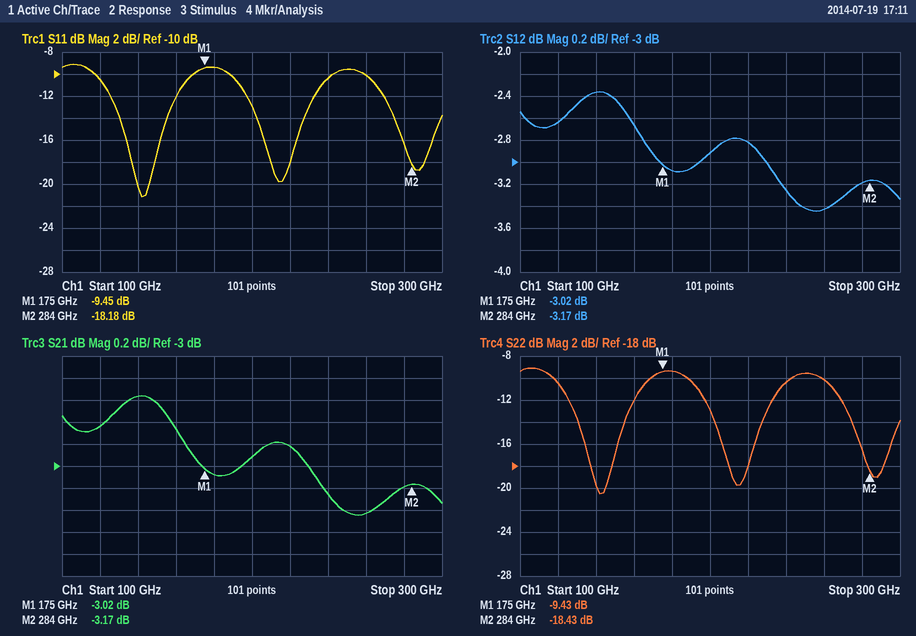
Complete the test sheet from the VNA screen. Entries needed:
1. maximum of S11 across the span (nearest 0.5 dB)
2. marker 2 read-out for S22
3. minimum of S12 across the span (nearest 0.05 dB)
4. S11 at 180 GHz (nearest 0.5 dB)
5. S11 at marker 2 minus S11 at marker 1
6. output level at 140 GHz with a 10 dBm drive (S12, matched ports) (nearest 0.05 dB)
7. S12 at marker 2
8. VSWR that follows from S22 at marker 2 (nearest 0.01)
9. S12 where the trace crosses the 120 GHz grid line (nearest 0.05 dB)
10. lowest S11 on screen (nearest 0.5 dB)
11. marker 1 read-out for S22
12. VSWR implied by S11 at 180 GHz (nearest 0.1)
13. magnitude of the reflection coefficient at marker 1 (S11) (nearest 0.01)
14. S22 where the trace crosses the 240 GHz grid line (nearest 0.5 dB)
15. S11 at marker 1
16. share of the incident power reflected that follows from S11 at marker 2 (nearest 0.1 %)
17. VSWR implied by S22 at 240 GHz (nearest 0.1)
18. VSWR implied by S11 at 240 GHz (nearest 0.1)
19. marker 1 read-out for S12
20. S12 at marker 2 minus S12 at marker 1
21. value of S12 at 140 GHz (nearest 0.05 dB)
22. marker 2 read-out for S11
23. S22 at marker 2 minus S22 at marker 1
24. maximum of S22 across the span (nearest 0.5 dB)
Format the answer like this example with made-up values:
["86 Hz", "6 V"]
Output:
["-9.0 dB", "-18.43 dB", "-3.45 dB", "-9.5 dB", "-8.73 dB", "7.65 dBm", "-3.17 dB", "1.27", "-2.65 dB", "-21.0 dB", "-9.43 dB", "2.0", "0.34", "-10.5 dB", "-9.45 dB", "1.5 %", "1.9", "1.9", "-3.02 dB", "-0.15 dB", "-2.35 dB", "-18.18 dB", "-9.00 dB", "-9.0 dB"]
